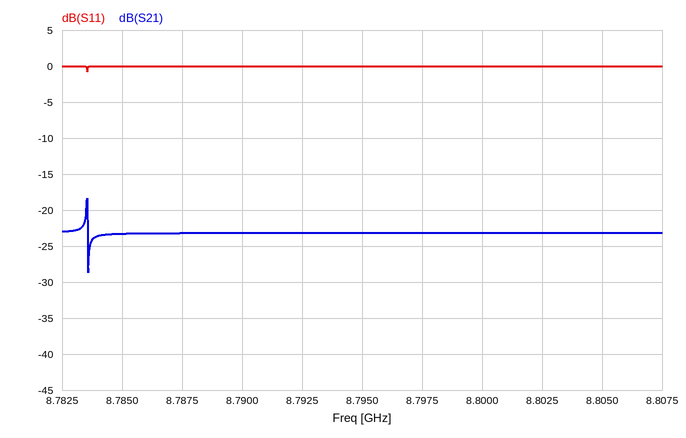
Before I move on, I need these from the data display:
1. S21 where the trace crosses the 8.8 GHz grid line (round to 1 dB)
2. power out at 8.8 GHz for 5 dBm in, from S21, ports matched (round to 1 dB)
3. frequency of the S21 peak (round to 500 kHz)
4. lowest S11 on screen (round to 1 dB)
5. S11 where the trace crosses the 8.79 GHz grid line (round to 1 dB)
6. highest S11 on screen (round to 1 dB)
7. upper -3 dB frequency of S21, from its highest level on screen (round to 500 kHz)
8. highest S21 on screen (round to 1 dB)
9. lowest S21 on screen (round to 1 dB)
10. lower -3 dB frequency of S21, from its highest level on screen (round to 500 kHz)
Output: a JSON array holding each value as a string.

["-23 dB", "-18 dBm", "8.7835 GHz", "-1 dB", "0 dB", "0 dB", "8.7835 GHz", "-18 dB", "-29 dB", "8.7835 GHz"]
